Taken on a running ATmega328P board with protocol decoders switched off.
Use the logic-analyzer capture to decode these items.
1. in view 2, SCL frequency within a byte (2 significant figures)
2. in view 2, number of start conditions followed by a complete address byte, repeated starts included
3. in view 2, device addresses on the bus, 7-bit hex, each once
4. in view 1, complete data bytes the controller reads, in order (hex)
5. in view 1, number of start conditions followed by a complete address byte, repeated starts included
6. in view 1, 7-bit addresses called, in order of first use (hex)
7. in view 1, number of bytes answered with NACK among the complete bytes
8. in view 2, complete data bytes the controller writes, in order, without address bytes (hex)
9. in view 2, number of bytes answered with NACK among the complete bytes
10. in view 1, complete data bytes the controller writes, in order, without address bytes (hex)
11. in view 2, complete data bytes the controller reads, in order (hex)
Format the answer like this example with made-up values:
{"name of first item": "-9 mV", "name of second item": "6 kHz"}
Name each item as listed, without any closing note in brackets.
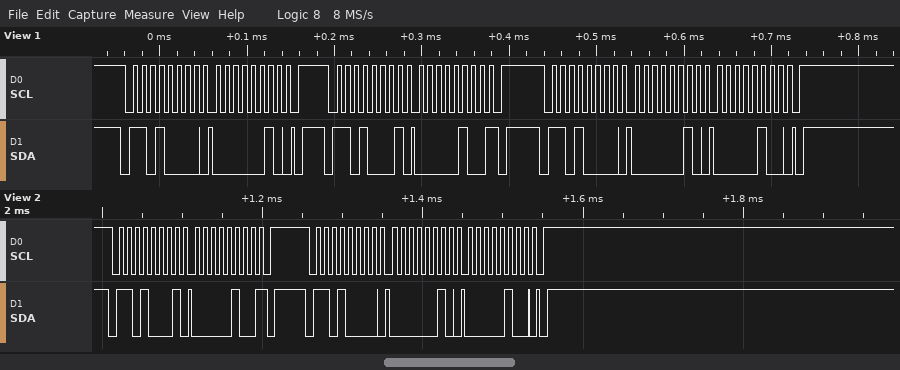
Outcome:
{"in view 2, SCL frequency within a byte": "100 kHz", "in view 2, number of start conditions followed by a complete address byte, repeated starts included": "2", "in view 2, device addresses on the bus, 7-bit hex, each once": "0x68", "in view 1, complete data bytes the controller reads, in order": "04", "in view 1, number of start conditions followed by a complete address byte, repeated starts included": "3", "in view 1, 7-bit addresses called, in order of first use": "0x68", "in view 1, number of bytes answered with NACK among the complete bytes": "1", "in view 2, complete data bytes the controller writes, in order, without address bytes": "02 04", "in view 2, number of bytes answered with NACK among the complete bytes": "1", "in view 1, complete data bytes the controller writes, in order, without address bytes": "02 02 04", "in view 2, complete data bytes the controller reads, in order": "04"}
